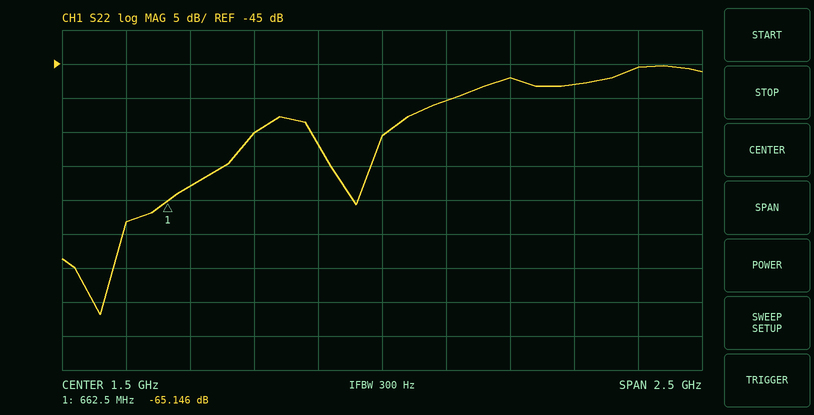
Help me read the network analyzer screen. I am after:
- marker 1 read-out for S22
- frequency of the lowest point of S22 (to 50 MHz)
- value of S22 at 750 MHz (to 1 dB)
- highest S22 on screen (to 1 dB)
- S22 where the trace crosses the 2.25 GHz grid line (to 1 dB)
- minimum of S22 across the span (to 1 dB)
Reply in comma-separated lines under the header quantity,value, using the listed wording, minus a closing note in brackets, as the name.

quantity,value
marker 1 read-out for S22,-65.146 dB
frequency of the lowest point of S22,400 MHz
value of S22 at 750 MHz,-63 dB
highest S22 on screen,-45 dB
S22 where the trace crosses the 2.25 GHz grid line,-48 dB
minimum of S22 across the span,-82 dB
